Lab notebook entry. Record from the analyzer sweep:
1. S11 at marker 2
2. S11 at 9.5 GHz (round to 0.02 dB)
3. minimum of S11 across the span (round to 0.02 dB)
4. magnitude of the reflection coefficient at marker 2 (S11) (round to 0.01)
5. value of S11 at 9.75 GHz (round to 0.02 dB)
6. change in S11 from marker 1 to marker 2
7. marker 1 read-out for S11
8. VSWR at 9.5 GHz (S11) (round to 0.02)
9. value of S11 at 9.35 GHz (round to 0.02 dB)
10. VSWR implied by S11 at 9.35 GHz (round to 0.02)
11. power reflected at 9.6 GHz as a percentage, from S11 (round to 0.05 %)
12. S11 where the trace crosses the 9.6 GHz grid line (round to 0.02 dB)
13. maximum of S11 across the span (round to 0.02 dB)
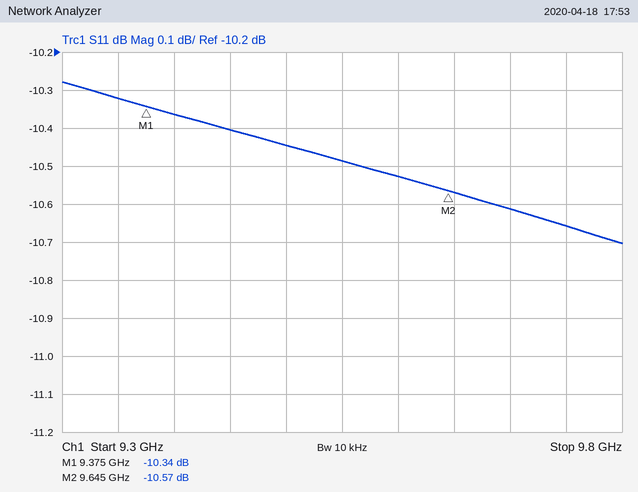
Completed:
-10.57 dB
-10.44 dB
-10.70 dB
0.30
-10.66 dB
-0.23 dB
-10.34 dB
1.86
-10.32 dB
1.88
8.85 %
-10.52 dB
-10.28 dB
